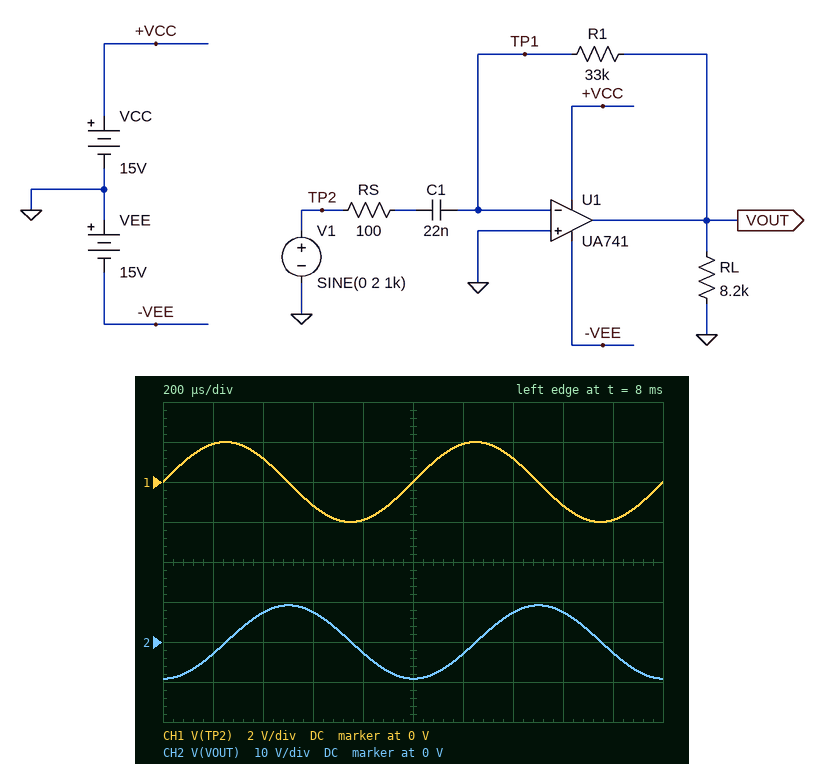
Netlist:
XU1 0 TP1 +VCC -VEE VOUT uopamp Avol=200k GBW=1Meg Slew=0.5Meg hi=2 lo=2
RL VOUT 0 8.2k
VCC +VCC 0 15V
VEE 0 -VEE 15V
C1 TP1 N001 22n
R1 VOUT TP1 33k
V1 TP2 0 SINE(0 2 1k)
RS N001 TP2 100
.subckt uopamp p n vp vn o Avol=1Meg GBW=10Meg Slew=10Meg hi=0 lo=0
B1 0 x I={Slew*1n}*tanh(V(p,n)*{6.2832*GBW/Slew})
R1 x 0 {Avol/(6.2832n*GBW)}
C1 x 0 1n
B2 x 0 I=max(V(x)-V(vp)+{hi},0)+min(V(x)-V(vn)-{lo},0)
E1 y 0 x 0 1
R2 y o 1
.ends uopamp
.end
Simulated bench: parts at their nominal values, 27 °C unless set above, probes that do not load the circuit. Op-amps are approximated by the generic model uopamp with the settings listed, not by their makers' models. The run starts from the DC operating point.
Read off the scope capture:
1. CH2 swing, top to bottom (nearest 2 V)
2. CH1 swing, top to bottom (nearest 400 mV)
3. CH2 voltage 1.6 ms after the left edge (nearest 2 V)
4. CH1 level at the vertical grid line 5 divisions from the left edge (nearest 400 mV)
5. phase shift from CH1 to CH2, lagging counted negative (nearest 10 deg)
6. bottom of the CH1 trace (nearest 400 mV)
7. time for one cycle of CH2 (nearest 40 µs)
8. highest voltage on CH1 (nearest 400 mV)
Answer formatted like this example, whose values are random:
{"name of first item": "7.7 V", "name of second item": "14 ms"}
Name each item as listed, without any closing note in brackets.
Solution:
{"CH2 swing, top to bottom": "18 V", "CH1 swing, top to bottom": "4.0 V", "CH2 voltage 1.6 ms after the left edge": "8 V", "CH1 level at the vertical grid line 5 divisions from the left edge": "0 V", "phase shift from CH1 to CH2, lagging counted negative": "-90 deg", "bottom of the CH1 trace": "-2.0 V", "time for one cycle of CH2": "1.00 ms", "highest voltage on CH1": "2.0 V"}
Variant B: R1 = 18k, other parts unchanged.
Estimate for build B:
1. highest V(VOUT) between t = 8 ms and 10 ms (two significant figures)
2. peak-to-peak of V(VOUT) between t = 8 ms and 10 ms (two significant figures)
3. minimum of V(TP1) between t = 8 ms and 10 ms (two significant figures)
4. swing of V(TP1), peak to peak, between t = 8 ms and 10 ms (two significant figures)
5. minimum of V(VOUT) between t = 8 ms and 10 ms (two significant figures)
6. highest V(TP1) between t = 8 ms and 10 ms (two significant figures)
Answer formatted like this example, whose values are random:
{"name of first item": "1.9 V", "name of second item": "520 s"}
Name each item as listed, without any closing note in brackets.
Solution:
{"highest V(VOUT) between t = 8 ms and 10 ms": "5.0 V", "peak-to-peak of V(VOUT) between t = 8 ms and 10 ms": "10 V", "minimum of V(TP1) between t = 8 ms and 10 ms": "-5.0 mV", "swing of V(TP1), peak to peak, between t = 8 ms and 10 ms": "10 mV", "minimum of V(VOUT) between t = 8 ms and 10 ms": "-5.0 V", "highest V(TP1) between t = 8 ms and 10 ms": "5.0 mV"}
